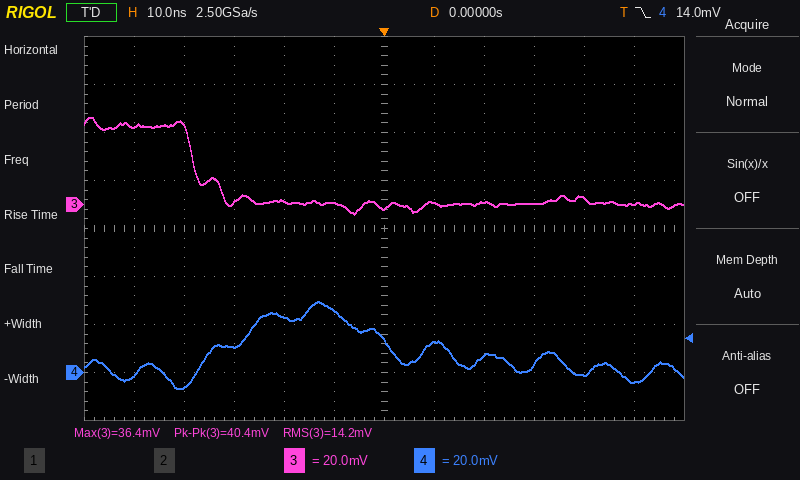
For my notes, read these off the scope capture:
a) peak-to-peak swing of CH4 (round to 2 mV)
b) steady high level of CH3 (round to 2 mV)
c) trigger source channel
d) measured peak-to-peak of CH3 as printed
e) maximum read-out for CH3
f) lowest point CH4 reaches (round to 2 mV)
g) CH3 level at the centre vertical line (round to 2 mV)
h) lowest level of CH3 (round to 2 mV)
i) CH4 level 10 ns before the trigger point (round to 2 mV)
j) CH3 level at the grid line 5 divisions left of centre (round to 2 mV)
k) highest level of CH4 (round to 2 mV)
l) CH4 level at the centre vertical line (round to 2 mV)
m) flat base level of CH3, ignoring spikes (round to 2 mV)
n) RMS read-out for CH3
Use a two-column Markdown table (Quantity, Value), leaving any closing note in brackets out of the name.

| Quantity | Value |
|---|---|
| peak-to-peak swing of CH4 | 36 mV |
| steady high level of CH3 | 32 mV |
| trigger source channel | CH4 |
| measured peak-to-peak of CH3 as printed | 40.4 mV |
| maximum read-out for CH3 | 36.4 mV |
| lowest point CH4 reaches | -6 mV |
| CH3 level at the centre vertical line | -2 mV |
| lowest level of CH3 | -4 mV |
| CH4 level 10 ns before the trigger point | 26 mV |
| CH3 level at the grid line 5 divisions left of centre | 32 mV |
| highest level of CH4 | 30 mV |
| CH4 level at the centre vertical line | 14 mV |
| flat base level of CH3, ignoring spikes | 0 mV |
| RMS read-out for CH3 | 14.2 mV |
